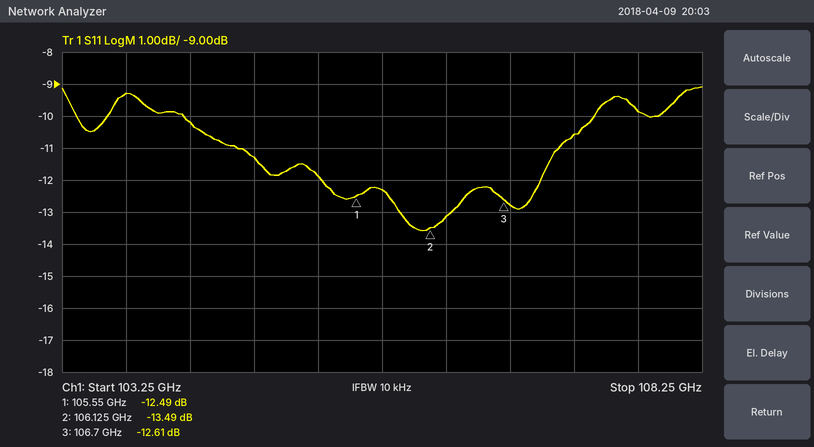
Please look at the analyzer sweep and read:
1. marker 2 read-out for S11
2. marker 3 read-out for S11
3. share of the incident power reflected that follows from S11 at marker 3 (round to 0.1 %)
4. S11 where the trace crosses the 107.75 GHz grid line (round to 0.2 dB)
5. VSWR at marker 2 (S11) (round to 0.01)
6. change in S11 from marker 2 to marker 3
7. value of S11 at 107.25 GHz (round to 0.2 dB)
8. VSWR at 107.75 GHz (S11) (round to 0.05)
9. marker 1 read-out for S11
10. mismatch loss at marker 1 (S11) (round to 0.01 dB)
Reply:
-13.49 dB
-12.61 dB
5.5 %
-9.8 dB
1.54
0.88 dB
-10.6 dB
1.95
-12.49 dB
0.25 dB
